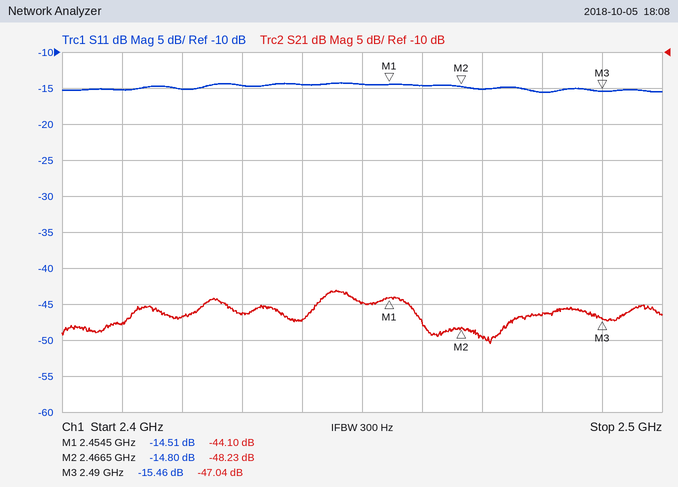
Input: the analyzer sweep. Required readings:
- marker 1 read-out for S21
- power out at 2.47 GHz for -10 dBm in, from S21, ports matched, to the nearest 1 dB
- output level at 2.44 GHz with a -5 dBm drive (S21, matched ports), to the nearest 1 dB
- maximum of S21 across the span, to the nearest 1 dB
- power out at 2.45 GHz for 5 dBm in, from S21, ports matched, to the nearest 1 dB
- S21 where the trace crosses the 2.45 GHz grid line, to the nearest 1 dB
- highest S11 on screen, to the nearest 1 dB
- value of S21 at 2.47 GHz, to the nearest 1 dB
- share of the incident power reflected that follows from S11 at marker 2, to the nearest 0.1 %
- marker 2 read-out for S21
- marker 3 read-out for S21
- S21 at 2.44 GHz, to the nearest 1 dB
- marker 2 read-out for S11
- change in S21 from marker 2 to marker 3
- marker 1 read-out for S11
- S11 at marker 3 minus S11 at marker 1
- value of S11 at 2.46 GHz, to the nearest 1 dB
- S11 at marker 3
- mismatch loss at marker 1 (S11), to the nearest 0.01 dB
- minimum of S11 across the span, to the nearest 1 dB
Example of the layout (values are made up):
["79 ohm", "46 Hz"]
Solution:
["-44.10 dB", "-60 dBm", "-52 dBm", "-43 dB", "-40 dBm", "-45 dB", "-14 dB", "-50 dB", "3.3 %", "-48.23 dB", "-47.04 dB", "-47 dB", "-14.80 dB", "1.19 dB", "-14.51 dB", "-0.95 dB", "-15 dB", "-15.46 dB", "0.16 dB", "-16 dB"]
